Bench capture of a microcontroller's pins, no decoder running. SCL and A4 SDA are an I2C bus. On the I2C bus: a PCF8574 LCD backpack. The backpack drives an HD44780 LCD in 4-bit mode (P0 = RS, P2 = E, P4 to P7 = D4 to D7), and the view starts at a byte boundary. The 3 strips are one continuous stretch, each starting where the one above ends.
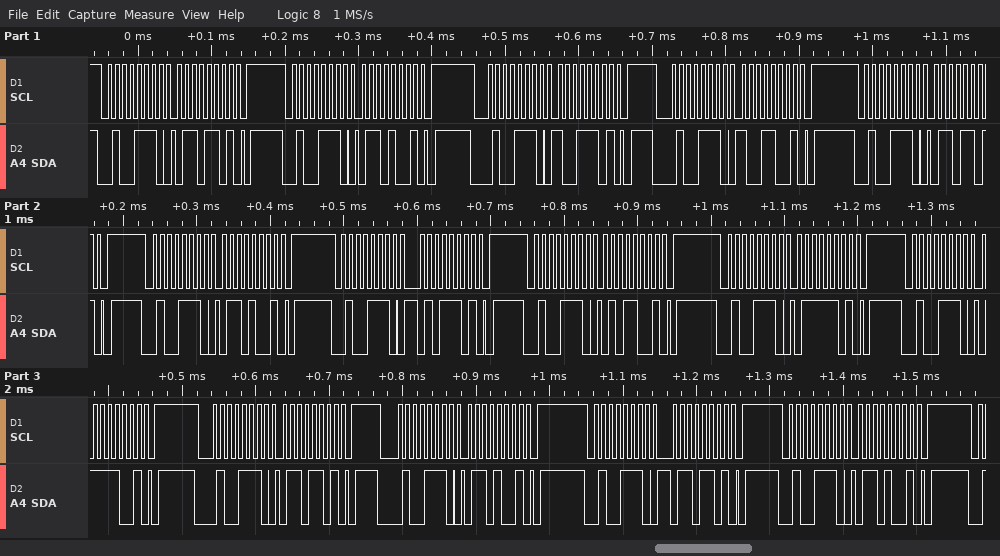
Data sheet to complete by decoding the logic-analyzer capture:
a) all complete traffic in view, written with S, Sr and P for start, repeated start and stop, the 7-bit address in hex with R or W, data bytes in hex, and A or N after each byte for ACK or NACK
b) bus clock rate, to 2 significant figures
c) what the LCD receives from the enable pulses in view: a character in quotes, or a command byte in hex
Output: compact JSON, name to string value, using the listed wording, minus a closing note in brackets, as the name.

{"all complete traffic in view, written with S, Sr and P for start, repeated start and stop, the 7-bit address in hex with R or W, data bytes in hex, and A or N after each byte for ACK or NACK": "S 27W A 6D A P S 27W A 69 A P S 27W A 9D A P S 27W A 99 A P S 27W A 6D A P S 27W A 69 A P S 27W A 5D A P S 27W A 59 A P S 27W A 7D A P S 27W A 79 A P S 27W A 6D A P S 27W A 69 A P S 27W A 6D A P S 27W A 69 A P", "bus clock rate, to 2 significant figures": "100 kHz", "what the LCD receives from the enable pulses in view: a character in quotes, or a command byte in hex": "'i' 'e' 'v'"}
